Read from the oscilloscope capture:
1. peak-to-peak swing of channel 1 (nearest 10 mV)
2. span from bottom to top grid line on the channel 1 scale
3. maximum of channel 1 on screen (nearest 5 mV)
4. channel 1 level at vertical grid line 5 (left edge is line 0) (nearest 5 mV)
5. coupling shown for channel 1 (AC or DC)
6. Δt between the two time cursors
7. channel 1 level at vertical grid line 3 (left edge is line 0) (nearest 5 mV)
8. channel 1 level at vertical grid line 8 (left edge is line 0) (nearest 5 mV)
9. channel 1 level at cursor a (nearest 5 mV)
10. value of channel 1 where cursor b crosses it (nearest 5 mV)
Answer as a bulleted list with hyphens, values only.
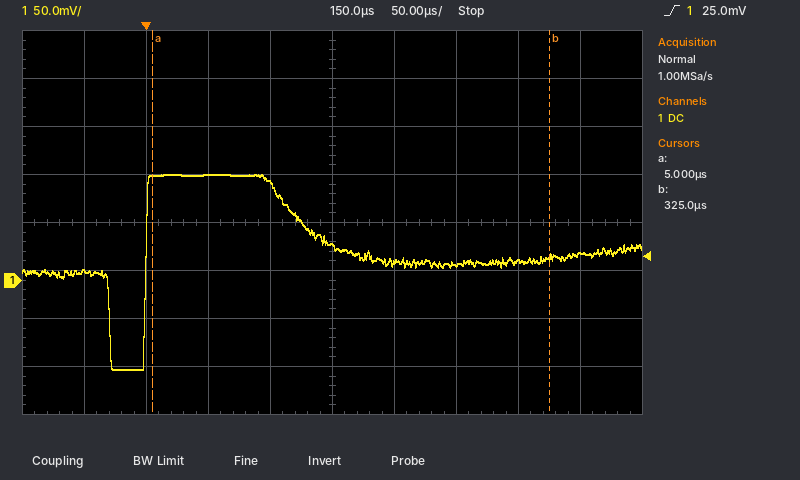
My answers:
- 200 mV
- 400 mV
- 110 mV
- 35 mV
- DC
- 320 µs
- 110 mV
- 20 mV
- 110 mV
- 25 mV
